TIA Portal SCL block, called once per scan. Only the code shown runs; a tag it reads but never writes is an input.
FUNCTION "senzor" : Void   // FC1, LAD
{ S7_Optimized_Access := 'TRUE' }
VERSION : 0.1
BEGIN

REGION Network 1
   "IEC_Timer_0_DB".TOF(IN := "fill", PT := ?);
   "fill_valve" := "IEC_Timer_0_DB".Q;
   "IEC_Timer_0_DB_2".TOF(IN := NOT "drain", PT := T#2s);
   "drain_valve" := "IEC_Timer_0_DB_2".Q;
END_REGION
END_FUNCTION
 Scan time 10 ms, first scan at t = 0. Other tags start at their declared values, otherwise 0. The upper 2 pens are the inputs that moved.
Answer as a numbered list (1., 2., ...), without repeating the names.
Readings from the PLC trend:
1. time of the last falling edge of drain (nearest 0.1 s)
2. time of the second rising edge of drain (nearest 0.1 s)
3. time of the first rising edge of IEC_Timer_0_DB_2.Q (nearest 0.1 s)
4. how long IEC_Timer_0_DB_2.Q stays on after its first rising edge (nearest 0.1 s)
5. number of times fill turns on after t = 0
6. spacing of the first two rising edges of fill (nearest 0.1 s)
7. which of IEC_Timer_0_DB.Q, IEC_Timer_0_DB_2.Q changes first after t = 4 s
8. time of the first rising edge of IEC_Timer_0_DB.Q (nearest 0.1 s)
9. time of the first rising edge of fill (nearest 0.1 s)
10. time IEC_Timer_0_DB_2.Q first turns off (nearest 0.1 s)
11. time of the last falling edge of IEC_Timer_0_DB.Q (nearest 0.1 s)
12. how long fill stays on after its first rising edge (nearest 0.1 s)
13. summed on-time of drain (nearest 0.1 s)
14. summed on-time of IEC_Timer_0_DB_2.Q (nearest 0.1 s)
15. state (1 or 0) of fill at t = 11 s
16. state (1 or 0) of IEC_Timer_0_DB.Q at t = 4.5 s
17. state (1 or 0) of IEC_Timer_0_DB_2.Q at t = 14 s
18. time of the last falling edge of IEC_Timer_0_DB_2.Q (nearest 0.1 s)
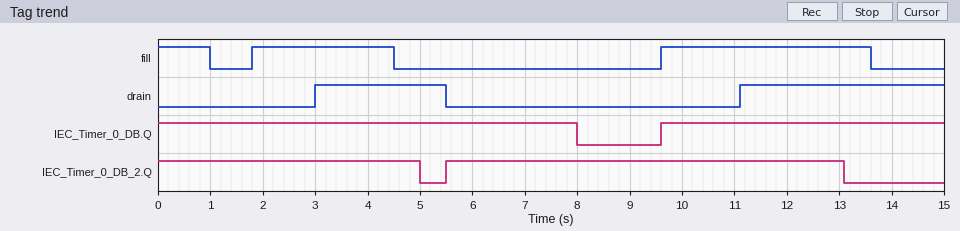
1. 5.5 s
2. 11.1 s
3. 5.5 s
4. 7.6 s
5. 2
6. 7.8 s
7. IEC_Timer_0_DB_2.Q
8. 9.6 s
9. 1.8 s
10. 5.0 s
11. 8.0 s
12. 2.7 s
13. 6.4 s
14. 12.6 s
15. 1
16. 1
17. 0
18. 13.1 s
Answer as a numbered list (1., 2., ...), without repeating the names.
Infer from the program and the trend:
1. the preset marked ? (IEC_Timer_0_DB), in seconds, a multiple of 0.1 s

1. 3.5 s
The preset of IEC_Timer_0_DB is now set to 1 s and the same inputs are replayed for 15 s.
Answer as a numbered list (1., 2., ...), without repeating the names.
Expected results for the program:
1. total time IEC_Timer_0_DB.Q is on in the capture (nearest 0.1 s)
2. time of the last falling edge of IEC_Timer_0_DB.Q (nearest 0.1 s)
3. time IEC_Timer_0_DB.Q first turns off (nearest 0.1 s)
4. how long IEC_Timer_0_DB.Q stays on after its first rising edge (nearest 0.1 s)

1. 10.5 s
2. 14.6 s
3. 5.5 s
4. 5.0 s
